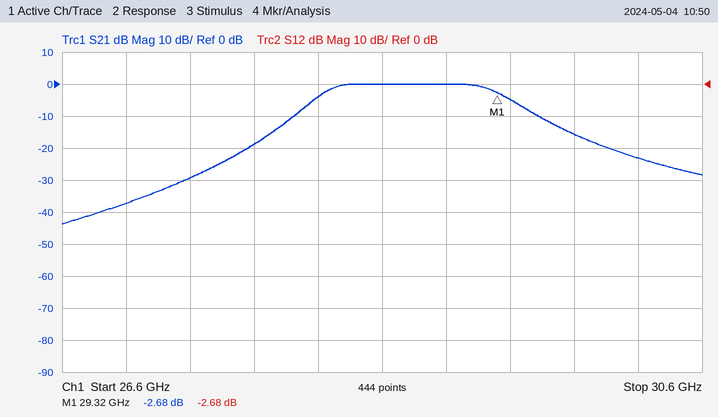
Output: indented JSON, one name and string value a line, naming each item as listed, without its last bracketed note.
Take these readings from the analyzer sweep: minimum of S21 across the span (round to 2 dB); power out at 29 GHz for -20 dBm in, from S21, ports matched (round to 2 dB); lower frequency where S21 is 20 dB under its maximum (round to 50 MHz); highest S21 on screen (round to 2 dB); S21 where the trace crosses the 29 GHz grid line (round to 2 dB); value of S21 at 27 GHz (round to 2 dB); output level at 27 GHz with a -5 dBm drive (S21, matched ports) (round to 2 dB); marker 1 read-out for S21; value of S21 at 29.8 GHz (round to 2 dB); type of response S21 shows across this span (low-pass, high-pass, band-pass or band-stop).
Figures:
{
  "minimum of S21 across the span": "-44 dB",
  "power out at 29 GHz for -20 dBm in, from S21, ports matched": "-20 dBm",
  "lower frequency where S21 is 20 dB under its maximum": "27.75 GHz",
  "highest S21 on screen": "0 dB",
  "S21 where the trace crosses the 29 GHz grid line": "0 dB",
  "value of S21 at 27 GHz": "-38 dB",
  "output level at 27 GHz with a -5 dBm drive (S21, matched ports)": "-42 dBm",
  "marker 1 read-out for S21": "-2.68 dB",
  "value of S21 at 29.8 GHz": "-16 dB",
  "type of response S21 shows across this span": "band-pass"
}
